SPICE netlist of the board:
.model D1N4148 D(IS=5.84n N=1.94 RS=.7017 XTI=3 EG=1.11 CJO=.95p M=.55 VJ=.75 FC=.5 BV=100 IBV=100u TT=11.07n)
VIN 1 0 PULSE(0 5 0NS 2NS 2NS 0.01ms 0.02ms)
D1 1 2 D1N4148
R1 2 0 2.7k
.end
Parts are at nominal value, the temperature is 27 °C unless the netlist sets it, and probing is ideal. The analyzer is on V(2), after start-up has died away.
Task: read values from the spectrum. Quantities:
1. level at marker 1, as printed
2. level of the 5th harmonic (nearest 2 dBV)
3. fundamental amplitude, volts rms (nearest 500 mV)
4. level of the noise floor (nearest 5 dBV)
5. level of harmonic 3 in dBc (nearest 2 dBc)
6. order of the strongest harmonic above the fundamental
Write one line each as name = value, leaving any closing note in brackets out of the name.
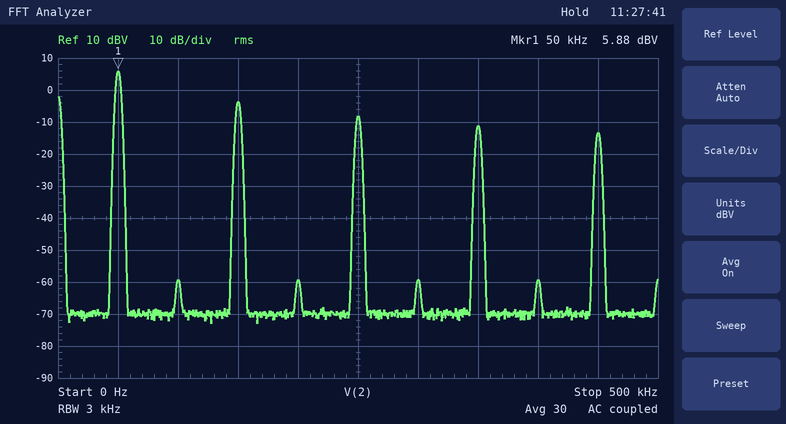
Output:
level at marker 1, as printed = 5.88 dBV
level of the 5th harmonic = -8 dBV
fundamental amplitude, volts rms = 2.0 V
level of the noise floor = -70 dBV
level of harmonic 3 in dBc = -10 dBc
order of the strongest harmonic above the fundamental = 3
